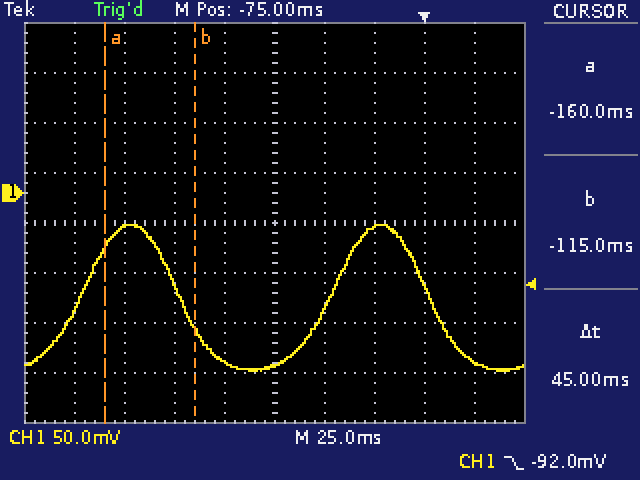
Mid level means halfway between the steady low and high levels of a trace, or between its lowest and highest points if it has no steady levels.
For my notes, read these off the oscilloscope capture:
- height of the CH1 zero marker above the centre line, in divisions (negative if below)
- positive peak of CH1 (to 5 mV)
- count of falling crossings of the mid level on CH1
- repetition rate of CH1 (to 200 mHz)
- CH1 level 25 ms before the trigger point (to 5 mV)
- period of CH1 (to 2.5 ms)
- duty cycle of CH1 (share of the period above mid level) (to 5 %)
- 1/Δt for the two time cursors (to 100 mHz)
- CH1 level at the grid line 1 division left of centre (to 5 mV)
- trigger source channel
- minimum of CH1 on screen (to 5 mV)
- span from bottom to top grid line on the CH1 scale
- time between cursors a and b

+0.6 div
-30 mV
2
8.0 Hz
-35 mV
125.0 ms
40 %
22.2 Hz
-170 mV
CH1
-180 mV
400 mV
45 ms
